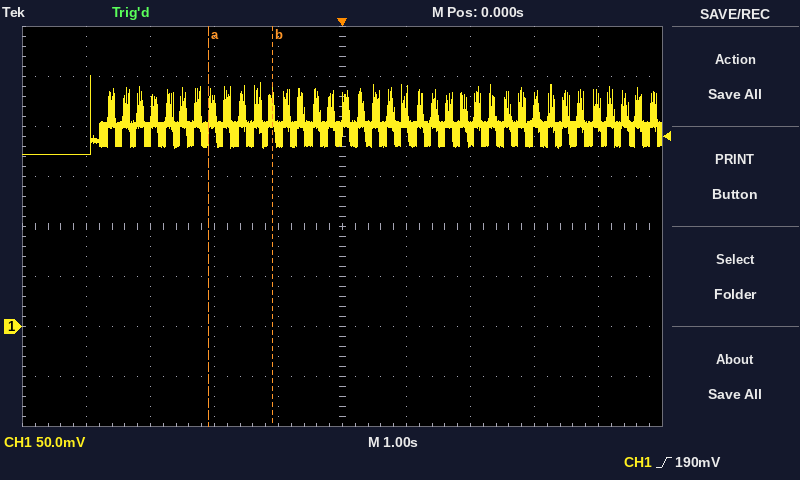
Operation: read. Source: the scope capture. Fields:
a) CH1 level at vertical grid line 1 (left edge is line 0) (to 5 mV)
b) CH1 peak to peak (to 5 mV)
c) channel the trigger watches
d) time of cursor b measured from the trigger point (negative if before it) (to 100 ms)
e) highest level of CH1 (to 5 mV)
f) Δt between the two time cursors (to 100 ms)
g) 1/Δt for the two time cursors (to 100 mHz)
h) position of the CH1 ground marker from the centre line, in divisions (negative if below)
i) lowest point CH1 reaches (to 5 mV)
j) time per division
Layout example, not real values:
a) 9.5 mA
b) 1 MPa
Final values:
a) 170 mV
b) 80 mV
c) CH1
d) -1.1 s
e) 250 mV
f) 1.0 s
g) 1.0 Hz
h) -2.0 div
i) 170 mV
j) 1 s
